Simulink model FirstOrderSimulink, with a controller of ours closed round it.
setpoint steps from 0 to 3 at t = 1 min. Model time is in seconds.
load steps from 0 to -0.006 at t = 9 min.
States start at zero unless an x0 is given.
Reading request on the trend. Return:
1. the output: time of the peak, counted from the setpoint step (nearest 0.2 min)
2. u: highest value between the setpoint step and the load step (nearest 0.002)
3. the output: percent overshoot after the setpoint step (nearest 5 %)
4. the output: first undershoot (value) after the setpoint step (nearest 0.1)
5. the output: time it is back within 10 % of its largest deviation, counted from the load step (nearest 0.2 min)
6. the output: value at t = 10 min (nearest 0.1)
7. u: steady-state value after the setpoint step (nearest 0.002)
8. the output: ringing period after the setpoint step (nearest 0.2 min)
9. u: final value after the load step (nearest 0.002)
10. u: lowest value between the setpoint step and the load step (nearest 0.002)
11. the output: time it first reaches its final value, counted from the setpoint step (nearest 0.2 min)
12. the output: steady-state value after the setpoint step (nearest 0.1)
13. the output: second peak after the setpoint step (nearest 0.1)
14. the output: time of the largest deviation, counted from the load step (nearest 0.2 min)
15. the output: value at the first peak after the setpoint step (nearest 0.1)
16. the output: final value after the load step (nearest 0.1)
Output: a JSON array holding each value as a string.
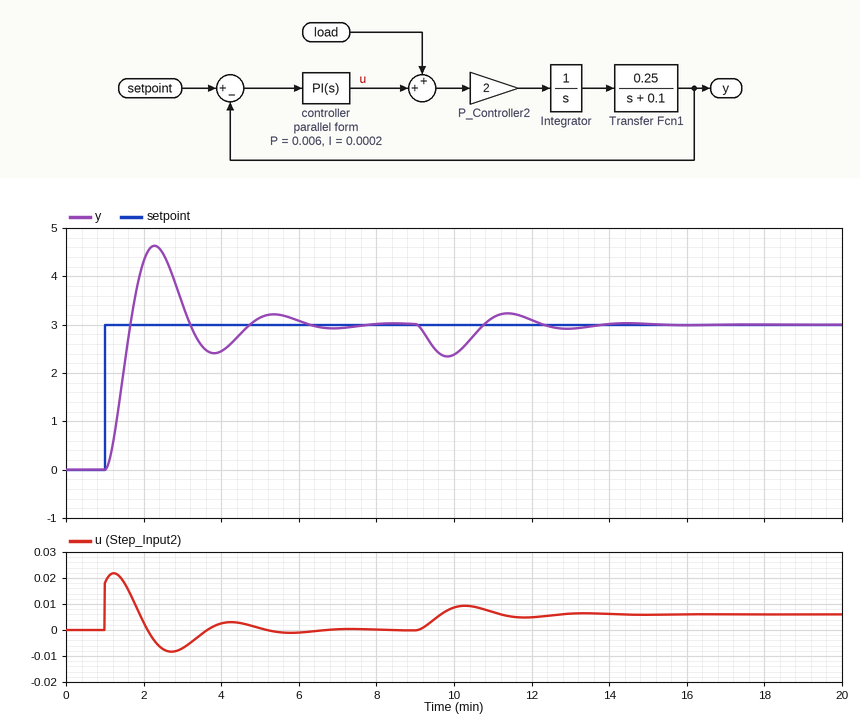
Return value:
["1.2 min", "0.022", "55 %", "2.4", "4.2 min", "2.4", "0.000", "3.0 min", "0.006", "-0.008", "0.6 min", "3.0", "3.2", "0.8 min", "4.6", "3.0"]
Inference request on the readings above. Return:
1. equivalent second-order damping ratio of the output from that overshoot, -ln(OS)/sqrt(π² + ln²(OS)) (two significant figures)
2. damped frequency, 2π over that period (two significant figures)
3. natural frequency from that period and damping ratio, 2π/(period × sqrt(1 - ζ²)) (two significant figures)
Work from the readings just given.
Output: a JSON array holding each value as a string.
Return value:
["0.19", "2.1 rad/min", "2.1 rad/min"]
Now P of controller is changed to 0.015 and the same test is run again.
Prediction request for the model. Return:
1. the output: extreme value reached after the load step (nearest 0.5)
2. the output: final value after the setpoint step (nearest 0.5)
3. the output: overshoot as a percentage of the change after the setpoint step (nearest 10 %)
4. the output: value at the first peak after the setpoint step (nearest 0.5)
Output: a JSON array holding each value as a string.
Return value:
["2.5", "3.0", "30 %", "4.0"]
